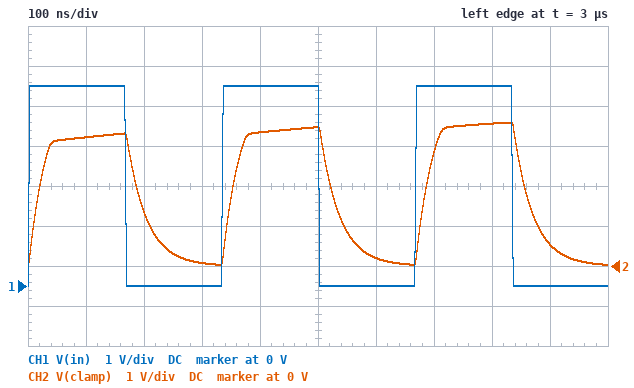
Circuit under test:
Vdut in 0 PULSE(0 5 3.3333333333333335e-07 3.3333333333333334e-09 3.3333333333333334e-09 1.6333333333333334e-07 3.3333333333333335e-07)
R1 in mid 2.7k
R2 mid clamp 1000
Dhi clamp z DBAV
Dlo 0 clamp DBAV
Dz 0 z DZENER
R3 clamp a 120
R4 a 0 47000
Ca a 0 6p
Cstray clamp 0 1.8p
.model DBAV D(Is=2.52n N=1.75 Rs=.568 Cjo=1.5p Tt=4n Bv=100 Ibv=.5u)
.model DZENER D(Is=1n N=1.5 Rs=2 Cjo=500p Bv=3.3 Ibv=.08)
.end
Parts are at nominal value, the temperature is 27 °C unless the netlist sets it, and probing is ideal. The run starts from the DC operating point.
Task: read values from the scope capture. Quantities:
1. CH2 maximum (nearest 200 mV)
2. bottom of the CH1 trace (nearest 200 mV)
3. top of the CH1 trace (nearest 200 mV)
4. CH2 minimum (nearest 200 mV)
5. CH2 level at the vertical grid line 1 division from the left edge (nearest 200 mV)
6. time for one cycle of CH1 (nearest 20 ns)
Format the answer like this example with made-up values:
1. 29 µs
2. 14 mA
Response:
1. 3.6 V
2. 0 V
3. 5.0 V
4. 0 V
5. 3.2 V
6. 340 ns
